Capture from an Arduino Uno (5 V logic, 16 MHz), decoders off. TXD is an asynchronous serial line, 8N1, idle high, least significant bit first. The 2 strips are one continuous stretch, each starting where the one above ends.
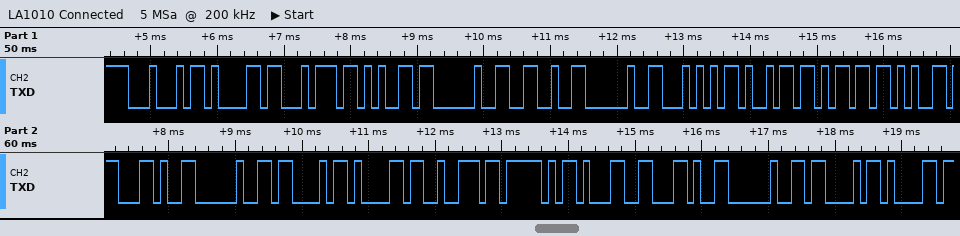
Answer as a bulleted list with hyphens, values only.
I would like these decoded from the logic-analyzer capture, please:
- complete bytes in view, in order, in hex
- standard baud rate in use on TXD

- 44 61 74 65 20 26 20 54 69 6D 65 2C 20 43 61 72 5F 31 2C 20 43 61
- 9600 baud
